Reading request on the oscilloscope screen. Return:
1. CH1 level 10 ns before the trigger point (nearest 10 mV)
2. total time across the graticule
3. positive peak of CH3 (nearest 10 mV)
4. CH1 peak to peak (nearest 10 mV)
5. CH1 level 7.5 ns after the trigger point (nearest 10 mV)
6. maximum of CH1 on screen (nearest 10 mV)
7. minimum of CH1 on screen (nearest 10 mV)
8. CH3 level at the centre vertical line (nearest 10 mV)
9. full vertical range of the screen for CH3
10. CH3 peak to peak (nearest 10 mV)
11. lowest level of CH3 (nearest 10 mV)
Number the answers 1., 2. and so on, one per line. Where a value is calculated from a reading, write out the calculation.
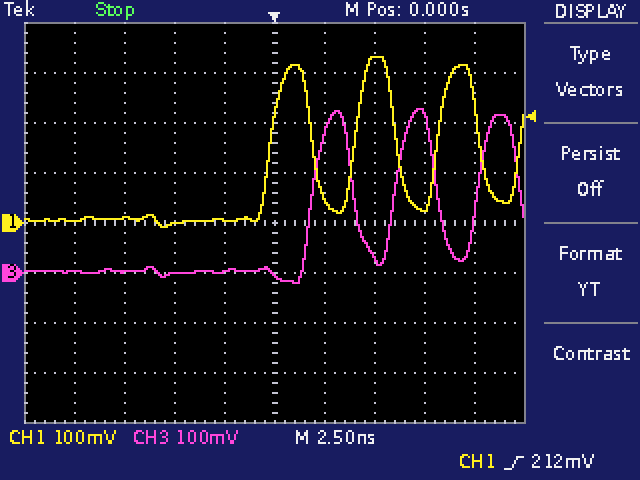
1. 0 mV
2. 25 ns
3. 330 mV
4. 330 mV − (-10 mV) = 340 mV
5. 30 mV
6. 330 mV
7. -10 mV
8. 0 mV
9. 800 mV
10. 330 mV − (-20 mV) = 350 mV
11. -20 mV
